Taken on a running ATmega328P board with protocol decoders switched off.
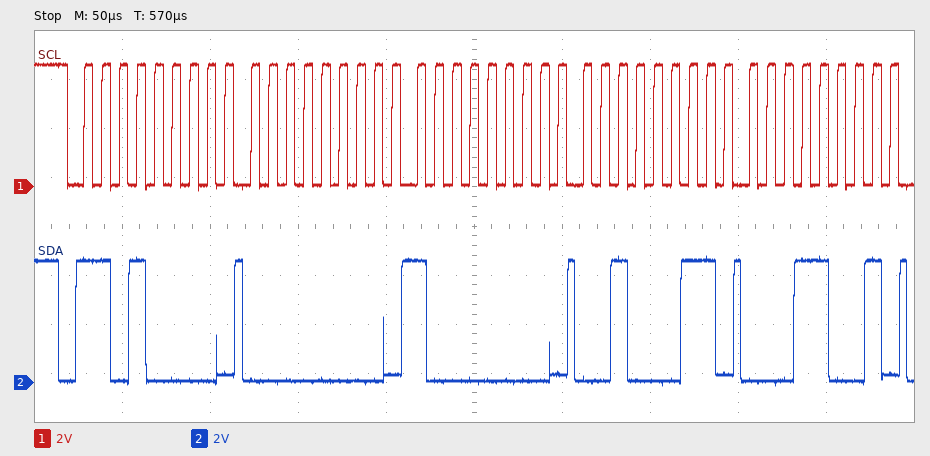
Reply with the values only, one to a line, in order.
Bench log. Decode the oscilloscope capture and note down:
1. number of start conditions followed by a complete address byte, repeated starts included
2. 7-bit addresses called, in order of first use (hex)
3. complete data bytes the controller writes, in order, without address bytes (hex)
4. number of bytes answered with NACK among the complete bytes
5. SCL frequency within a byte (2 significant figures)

1
0x68
00 80 23 19
0
100 kHz
